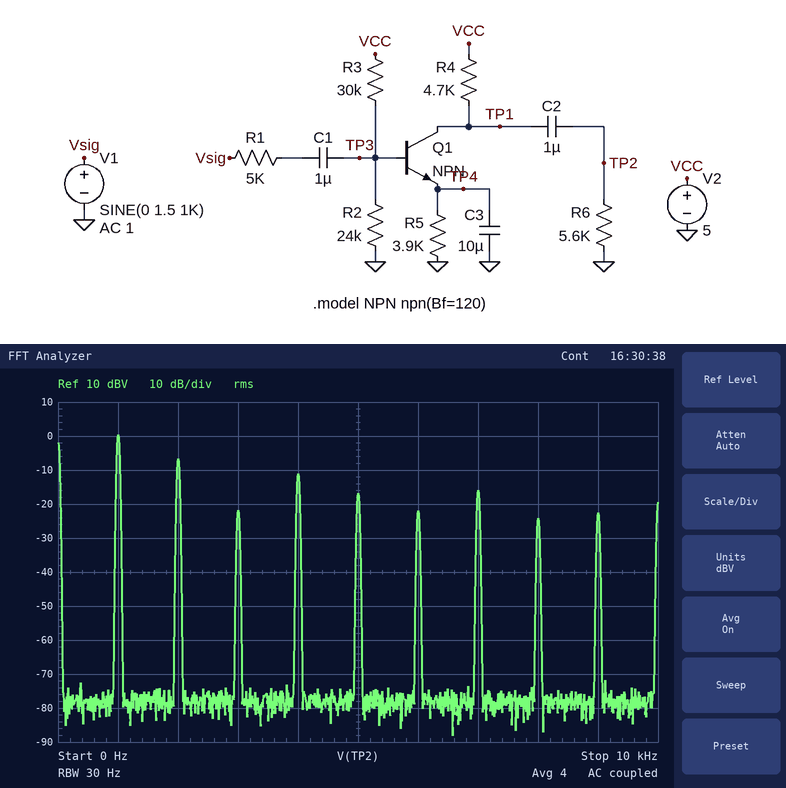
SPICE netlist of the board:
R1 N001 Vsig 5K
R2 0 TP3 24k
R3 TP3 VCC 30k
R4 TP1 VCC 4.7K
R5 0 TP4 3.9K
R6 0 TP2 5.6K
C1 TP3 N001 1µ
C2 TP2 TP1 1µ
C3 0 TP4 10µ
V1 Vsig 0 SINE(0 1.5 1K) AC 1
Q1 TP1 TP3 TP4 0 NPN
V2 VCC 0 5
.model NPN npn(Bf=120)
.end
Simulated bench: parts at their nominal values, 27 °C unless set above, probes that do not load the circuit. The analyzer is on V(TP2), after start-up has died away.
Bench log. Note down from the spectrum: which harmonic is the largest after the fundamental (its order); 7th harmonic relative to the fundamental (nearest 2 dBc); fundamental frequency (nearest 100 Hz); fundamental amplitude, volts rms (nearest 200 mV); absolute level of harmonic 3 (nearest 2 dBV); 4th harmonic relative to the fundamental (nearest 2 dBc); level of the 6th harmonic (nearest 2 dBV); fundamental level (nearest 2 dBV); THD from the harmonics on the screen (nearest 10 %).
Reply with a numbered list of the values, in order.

1. 2
2. -16 dBc
3. 1.0 kHz
4. 1.0 V
5. -22 dBV
6. -12 dBc
7. -22 dBV
8. 0 dBV
9. 60 %
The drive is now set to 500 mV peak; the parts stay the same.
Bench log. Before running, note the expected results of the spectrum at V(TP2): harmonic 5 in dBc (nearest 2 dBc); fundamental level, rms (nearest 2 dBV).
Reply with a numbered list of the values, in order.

1. -18 dBc
2. 0 dBV
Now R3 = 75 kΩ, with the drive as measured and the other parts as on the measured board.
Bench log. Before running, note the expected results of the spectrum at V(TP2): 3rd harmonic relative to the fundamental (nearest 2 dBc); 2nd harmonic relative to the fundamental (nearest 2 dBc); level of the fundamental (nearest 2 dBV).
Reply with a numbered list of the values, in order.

1. -8 dBc
2. -2 dBc
3. 0 dBV
